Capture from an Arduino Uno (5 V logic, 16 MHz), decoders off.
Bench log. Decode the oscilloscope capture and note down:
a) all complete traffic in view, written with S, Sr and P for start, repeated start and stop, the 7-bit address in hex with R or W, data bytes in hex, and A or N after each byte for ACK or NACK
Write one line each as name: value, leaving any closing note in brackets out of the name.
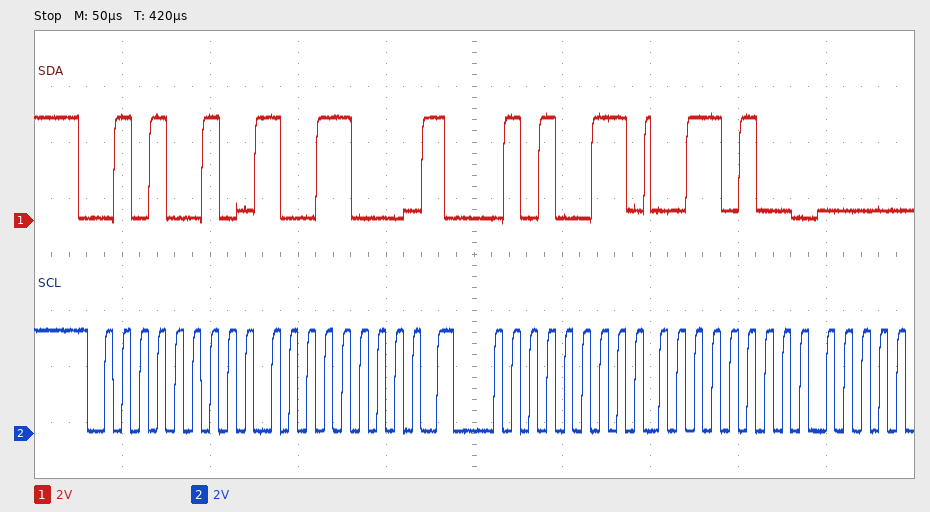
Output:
all complete traffic in view, written with S, Sr and P for start, repeated start and stop, the 7-bit address in hex with R or W, data bytes in hex, and A or N after each byte for ACK or NACK: S 29W A 98 A Sr 29R A 34 A
